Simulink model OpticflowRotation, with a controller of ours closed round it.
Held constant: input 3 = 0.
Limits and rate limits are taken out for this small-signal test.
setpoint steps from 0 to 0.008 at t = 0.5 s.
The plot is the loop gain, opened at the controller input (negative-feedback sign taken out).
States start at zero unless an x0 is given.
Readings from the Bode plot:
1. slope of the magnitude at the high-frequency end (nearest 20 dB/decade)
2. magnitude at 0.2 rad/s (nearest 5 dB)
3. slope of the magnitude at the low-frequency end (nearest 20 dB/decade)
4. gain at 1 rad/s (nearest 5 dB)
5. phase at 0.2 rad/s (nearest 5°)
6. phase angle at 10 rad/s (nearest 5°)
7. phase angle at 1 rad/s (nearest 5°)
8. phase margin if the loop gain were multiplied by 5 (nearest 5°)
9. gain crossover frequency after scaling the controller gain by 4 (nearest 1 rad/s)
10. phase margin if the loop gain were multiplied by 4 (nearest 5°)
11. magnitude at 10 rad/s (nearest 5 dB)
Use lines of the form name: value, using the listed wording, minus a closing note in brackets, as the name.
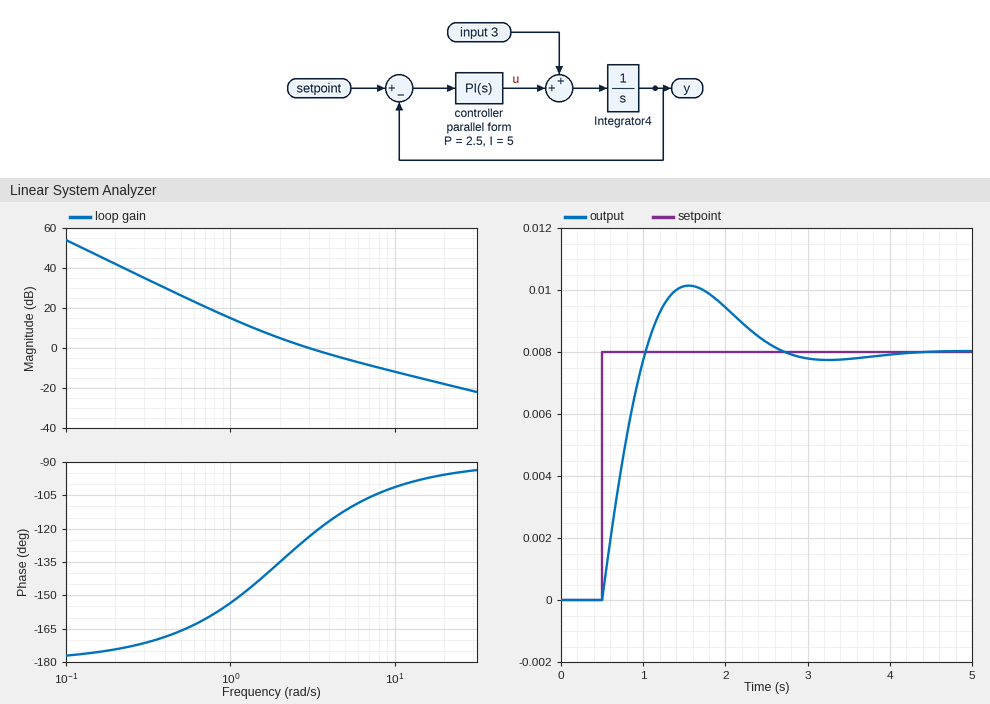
slope of the magnitude at the high-frequency end: -20 dB/decade
magnitude at 0.2 rad/s: 40 dB
slope of the magnitude at the low-frequency end: -40 dB/decade
gain at 1 rad/s: 15 dB
phase at 0.2 rad/s: -175°
phase angle at 10 rad/s: -100°
phase angle at 1 rad/s: -155°
phase margin if the loop gain were multiplied by 5: 80°
gain crossover frequency after scaling the controller gain by 4: 10 rad/s
phase margin if the loop gain were multiplied by 4: 80°
magnitude at 10 rad/s: -10 dB
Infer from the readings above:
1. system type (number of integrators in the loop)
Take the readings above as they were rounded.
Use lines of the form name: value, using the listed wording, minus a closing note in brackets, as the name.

system type: 2
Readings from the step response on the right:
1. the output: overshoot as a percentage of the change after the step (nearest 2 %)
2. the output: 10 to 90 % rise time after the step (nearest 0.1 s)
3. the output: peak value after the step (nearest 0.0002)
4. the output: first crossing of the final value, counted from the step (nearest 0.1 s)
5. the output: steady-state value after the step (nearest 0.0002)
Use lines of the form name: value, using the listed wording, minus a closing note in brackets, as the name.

the output: overshoot as a percentage of the change after the step: 26 %
the output: 10 to 90 % rise time after the step: 0.4 s
the output: peak value after the step: 0.0102
the output: first crossing of the final value, counted from the step: 0.5 s
the output: steady-state value after the step: 0.0080
